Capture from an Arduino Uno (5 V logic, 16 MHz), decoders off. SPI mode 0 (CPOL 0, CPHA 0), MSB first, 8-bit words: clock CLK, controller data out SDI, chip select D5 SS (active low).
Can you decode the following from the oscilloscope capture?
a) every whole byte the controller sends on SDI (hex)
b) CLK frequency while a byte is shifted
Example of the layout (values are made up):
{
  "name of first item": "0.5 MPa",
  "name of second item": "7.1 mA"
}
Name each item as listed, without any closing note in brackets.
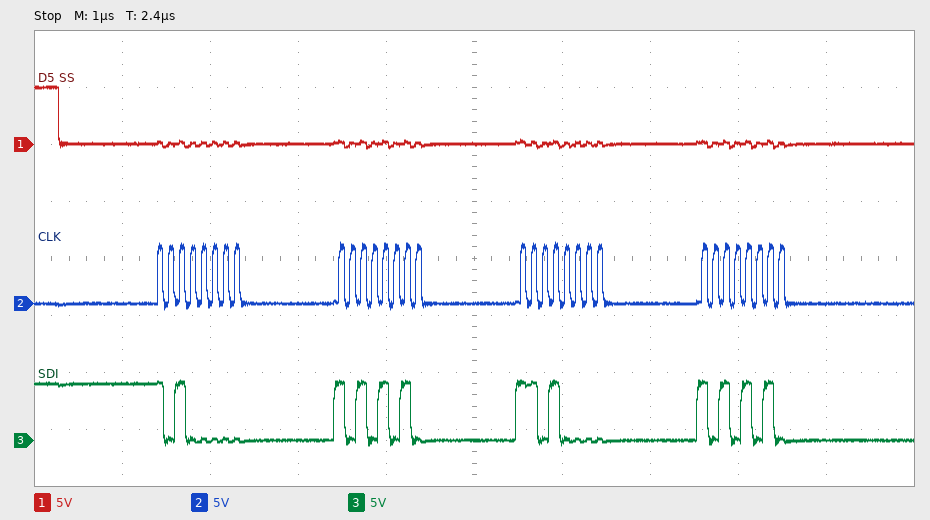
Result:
{
  "every whole byte the controller sends on SDI": "A0 AA D0 AA",
  "CLK frequency while a byte is shifted": "8 MHz"
}
